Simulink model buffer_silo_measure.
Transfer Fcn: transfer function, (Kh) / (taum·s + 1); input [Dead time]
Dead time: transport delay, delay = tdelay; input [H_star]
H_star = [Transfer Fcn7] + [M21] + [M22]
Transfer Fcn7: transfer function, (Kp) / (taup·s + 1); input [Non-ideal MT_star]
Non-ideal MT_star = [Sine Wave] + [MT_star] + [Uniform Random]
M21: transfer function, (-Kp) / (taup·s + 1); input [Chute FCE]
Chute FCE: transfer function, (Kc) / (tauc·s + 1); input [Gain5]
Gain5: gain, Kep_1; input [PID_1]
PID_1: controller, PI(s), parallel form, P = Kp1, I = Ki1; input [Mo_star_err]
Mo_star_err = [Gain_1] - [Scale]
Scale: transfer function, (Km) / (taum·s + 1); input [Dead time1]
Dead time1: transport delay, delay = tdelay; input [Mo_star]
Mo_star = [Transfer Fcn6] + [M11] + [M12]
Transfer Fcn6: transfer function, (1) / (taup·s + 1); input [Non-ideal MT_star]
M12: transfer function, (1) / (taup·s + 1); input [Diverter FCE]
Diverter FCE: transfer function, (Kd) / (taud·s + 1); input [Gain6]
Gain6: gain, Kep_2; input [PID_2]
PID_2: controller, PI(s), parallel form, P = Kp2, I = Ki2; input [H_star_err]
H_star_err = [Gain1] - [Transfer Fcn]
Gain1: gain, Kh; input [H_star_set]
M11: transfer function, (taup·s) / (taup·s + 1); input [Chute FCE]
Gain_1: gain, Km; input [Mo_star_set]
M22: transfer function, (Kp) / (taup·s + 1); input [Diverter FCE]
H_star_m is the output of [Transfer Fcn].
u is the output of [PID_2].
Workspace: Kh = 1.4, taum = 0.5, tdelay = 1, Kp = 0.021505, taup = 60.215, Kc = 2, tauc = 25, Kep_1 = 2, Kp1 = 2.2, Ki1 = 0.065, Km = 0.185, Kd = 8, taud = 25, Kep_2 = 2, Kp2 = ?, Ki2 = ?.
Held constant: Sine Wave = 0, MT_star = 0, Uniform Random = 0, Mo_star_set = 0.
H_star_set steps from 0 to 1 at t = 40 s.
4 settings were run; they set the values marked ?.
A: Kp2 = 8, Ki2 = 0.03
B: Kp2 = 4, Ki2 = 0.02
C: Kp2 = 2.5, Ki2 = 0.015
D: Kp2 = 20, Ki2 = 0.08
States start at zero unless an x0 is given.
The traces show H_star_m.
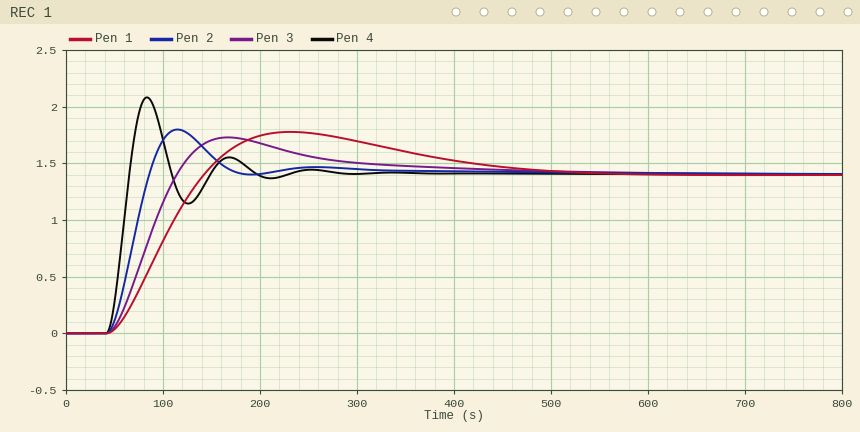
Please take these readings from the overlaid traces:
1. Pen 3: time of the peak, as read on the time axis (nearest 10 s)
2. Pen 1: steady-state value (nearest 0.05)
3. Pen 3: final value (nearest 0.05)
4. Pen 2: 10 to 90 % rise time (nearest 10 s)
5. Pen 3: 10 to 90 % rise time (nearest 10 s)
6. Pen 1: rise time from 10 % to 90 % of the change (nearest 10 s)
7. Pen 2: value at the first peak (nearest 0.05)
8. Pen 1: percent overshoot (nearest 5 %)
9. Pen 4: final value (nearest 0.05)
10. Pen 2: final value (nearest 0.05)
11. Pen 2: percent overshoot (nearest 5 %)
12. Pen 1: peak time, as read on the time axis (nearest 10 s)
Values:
170 s
1.40
1.40
30 s
50 s
70 s
1.80
25 %
1.40
1.40
30 %
230 s
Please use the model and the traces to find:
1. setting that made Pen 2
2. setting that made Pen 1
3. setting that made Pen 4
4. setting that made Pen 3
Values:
A
C
D
B
